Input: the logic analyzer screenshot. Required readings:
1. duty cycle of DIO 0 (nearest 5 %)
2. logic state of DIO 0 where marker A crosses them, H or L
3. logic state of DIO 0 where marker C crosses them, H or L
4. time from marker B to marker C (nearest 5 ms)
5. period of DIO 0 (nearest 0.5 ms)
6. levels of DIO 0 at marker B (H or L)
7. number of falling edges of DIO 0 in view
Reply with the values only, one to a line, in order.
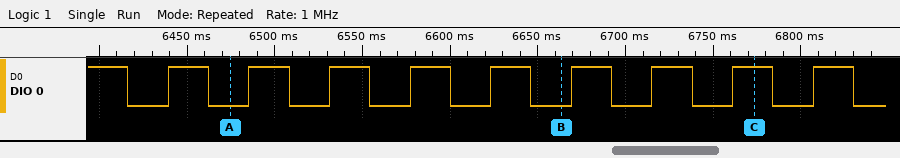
50 %
DIO 0=L
DIO 0=H
110 ms
46 ms
DIO 0=L
10
